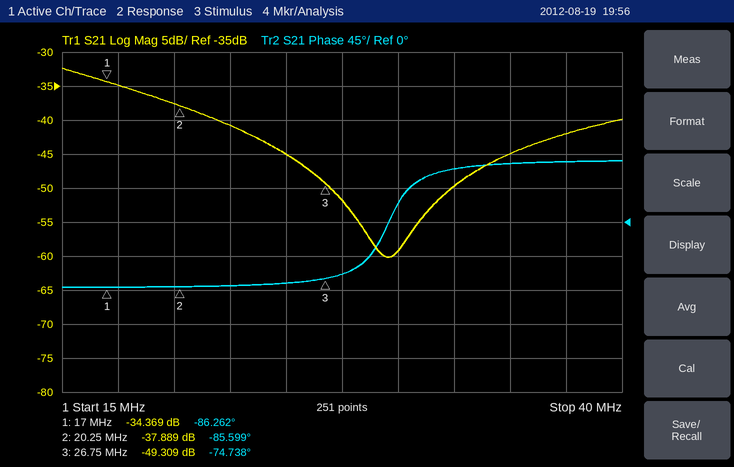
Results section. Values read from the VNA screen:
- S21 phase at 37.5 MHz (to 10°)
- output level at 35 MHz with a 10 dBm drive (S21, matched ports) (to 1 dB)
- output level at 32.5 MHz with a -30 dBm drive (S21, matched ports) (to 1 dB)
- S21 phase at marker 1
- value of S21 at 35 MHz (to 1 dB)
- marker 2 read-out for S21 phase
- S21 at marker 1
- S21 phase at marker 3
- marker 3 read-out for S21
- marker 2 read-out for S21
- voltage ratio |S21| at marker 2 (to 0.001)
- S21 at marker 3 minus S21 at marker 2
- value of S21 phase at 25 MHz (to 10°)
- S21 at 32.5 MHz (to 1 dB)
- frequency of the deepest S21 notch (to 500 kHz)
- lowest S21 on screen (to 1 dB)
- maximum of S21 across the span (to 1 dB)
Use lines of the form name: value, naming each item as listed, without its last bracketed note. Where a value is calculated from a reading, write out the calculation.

S21 phase at 37.5 MHz: 80°
output level at 35 MHz with a 10 dBm drive (S21, matched ports): 10 dBm + (-45 dB) = -35 dBm
output level at 32.5 MHz with a -30 dBm drive (S21, matched ports): -30 dBm + (-50 dB) = -80 dBm
S21 phase at marker 1: -86.262°
value of S21 at 35 MHz: -45 dB
marker 2 read-out for S21 phase: -85.599°
S21 at marker 1: -34.369 dB
S21 phase at marker 3: -74.738°
marker 3 read-out for S21: -49.309 dB
marker 2 read-out for S21: -37.889 dB
voltage ratio |S21| at marker 2: 10^(-37.889/20) ≈ 0.013
S21 at marker 3 minus S21 at marker 2: -49.309 − (-37.889) = -11.420 dB
value of S21 phase at 25 MHz: -80°
S21 at 32.5 MHz: -50 dB
frequency of the deepest S21 notch: 29.5 MHz
lowest S21 on screen: -60 dB
maximum of S21 across the span: -32 dB
